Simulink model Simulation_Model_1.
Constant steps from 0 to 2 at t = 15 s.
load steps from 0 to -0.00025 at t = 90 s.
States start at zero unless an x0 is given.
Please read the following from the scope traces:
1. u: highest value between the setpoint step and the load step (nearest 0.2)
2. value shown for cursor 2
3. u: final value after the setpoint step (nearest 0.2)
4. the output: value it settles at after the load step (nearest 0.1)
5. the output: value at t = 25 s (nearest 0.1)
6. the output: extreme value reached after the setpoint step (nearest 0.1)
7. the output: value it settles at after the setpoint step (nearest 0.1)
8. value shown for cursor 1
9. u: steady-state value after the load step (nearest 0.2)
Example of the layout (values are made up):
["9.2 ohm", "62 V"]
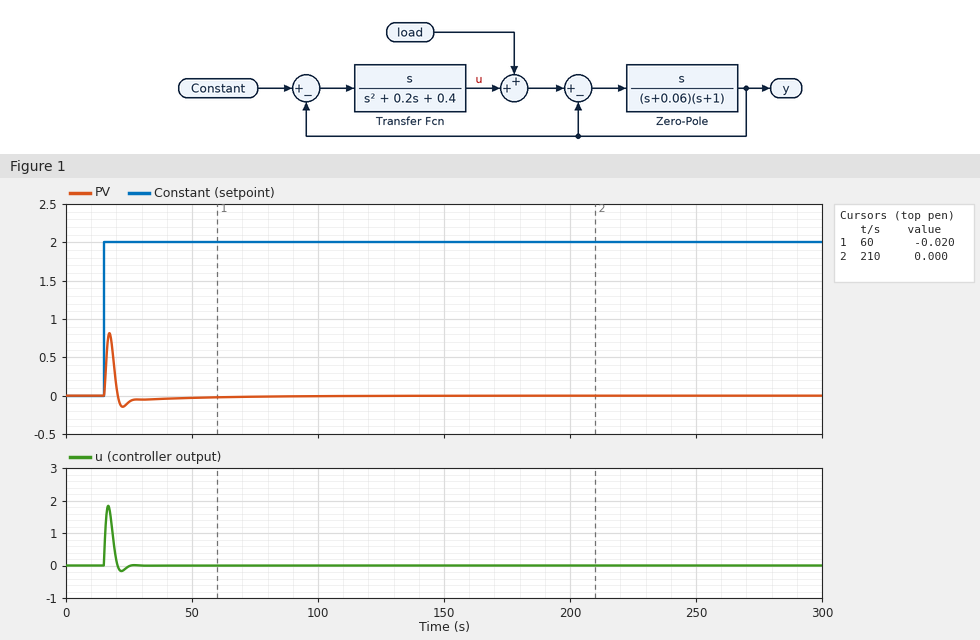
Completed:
["1.8", "0.000", "0.0", "0.0", "-0.1", "0.8", "0.0", "-0.020", "0.0"]
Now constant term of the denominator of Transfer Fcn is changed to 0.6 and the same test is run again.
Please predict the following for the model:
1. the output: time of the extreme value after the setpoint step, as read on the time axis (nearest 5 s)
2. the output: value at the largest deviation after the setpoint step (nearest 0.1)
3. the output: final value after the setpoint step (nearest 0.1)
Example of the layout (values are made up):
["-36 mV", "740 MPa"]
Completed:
["15 s", "0.7", "0.0"]
